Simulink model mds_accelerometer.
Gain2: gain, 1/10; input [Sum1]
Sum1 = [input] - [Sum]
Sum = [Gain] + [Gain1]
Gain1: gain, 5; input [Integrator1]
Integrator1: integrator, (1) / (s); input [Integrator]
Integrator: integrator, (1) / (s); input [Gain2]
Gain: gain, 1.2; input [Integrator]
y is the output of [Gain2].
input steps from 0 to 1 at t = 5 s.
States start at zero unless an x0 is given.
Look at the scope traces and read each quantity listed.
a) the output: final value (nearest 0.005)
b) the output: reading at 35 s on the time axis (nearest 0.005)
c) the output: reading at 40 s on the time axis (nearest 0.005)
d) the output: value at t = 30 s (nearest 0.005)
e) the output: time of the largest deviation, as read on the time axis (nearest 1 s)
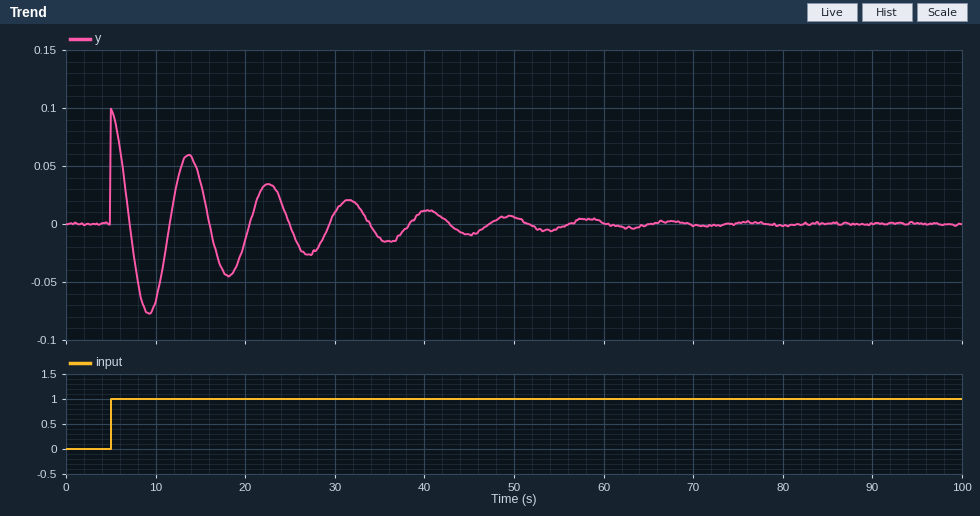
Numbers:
0.000
-0.010
0.010
0.010
5 s
